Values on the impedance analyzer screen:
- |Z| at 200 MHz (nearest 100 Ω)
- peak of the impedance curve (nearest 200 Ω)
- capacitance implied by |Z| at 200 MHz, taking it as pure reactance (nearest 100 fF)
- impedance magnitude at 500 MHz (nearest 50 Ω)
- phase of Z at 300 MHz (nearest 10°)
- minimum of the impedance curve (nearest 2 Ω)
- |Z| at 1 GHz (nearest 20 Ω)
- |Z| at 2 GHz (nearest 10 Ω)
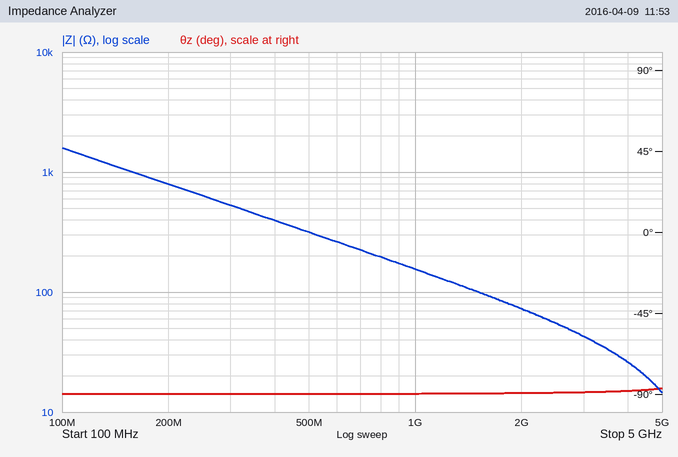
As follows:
800 Ω
1.6 kΩ
1.0 pF
300 Ω
-90°
14 Ω
160 Ω
70 Ω
